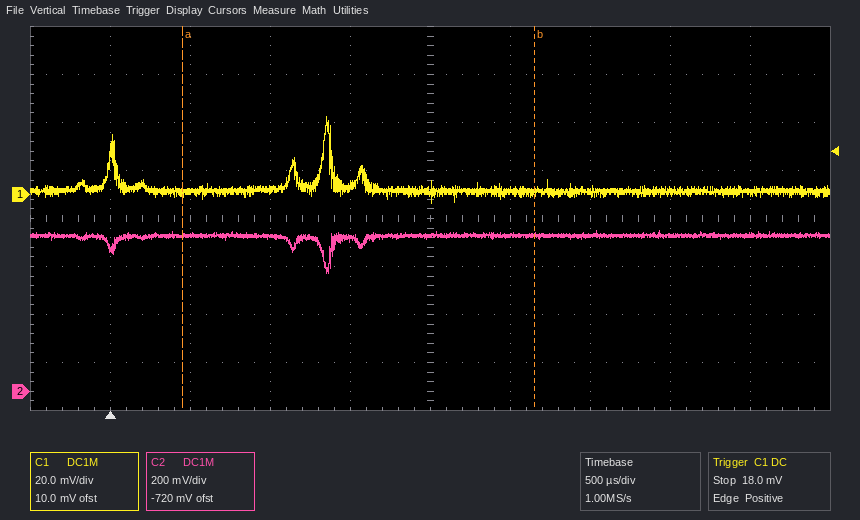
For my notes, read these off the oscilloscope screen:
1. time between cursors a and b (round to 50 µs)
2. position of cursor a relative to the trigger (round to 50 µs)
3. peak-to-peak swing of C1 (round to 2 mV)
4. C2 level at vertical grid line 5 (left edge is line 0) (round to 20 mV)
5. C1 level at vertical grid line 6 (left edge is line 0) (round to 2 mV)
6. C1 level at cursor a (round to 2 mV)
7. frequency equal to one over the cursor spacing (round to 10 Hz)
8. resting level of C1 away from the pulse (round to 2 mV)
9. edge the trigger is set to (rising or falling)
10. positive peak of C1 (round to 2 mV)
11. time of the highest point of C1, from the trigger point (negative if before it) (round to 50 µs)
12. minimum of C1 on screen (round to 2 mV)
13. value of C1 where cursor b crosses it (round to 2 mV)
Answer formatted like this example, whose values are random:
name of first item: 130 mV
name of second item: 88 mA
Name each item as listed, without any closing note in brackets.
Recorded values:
time between cursors a and b: 2.20 ms
position of cursor a relative to the trigger: +450 µs
peak-to-peak swing of C1: 36 mV
C2 level at vertical grid line 5 (left edge is line 0): 640 mV
C1 level at vertical grid line 6 (left edge is line 0): 2 mV
C1 level at cursor a: 0 mV
frequency equal to one over the cursor spacing: 450 Hz
resting level of C1 away from the pulse: 2 mV
edge the trigger is set to: rising
positive peak of C1: 32 mV
time of the highest point of C1, from the trigger point (negative if before it): +1.35 ms
minimum of C1 on screen: -4 mV
value of C1 where cursor b crosses it: 2 mV
